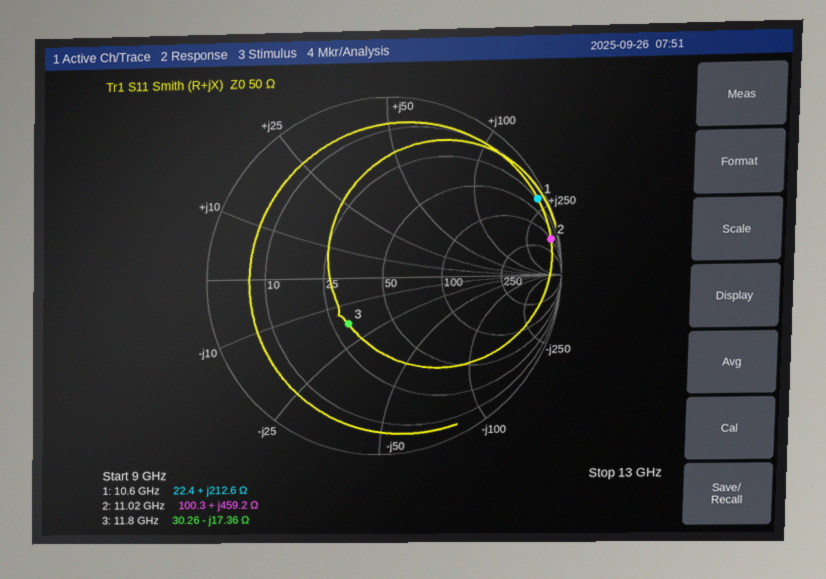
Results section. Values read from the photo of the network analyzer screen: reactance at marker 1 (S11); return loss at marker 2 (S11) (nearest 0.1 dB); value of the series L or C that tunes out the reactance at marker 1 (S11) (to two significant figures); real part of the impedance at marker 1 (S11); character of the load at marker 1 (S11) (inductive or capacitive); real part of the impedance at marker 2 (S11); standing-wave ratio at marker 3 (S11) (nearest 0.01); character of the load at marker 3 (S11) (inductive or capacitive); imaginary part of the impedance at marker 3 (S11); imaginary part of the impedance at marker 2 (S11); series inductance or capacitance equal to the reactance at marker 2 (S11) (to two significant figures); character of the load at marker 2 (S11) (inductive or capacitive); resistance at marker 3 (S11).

+212.6 Ω
0.4 dB
71 fF
22.4 Ω
inductive
100.3 Ω
1.94
capacitive
-17.36 Ω
+459.2 Ω
6.6 nH
inductive
30.26 Ω
